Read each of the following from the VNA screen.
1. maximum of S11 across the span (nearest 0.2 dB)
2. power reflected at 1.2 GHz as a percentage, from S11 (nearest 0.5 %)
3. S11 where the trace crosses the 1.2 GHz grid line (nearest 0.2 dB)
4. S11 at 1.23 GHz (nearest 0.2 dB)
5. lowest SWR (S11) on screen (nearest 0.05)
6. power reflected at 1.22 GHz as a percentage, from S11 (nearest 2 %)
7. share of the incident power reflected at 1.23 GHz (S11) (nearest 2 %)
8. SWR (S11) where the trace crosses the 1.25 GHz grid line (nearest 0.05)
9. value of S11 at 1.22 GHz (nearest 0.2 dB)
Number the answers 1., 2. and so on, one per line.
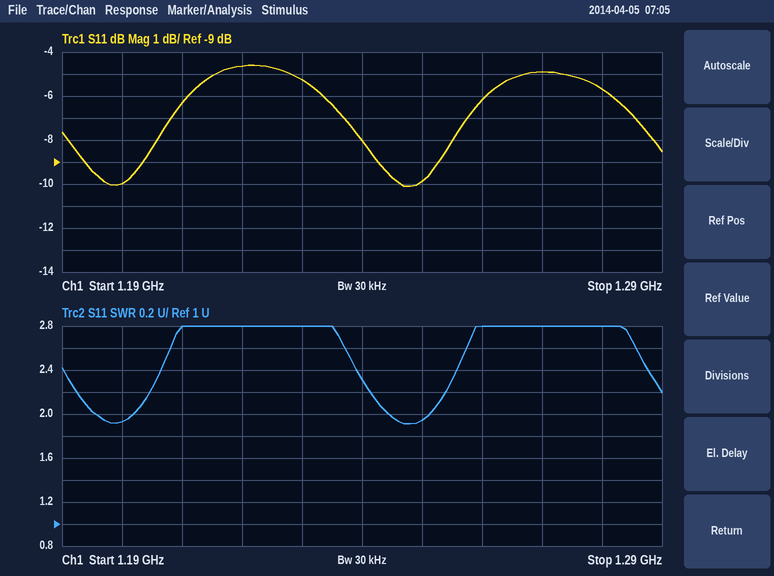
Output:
1. -4.6 dB
2. 10.0 %
3. -10.0 dB
4. -5.2 dB
5. 1.90
6. 34 %
7. 30 %
8. 1.95
9. -4.6 dB
